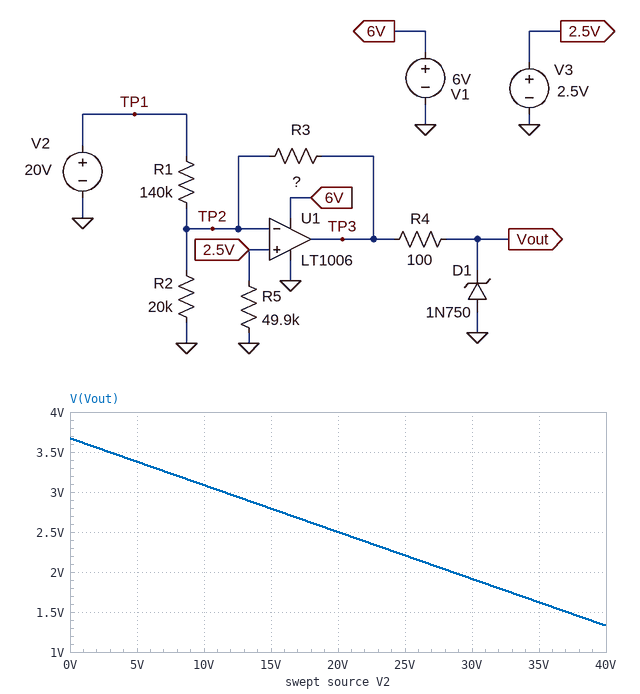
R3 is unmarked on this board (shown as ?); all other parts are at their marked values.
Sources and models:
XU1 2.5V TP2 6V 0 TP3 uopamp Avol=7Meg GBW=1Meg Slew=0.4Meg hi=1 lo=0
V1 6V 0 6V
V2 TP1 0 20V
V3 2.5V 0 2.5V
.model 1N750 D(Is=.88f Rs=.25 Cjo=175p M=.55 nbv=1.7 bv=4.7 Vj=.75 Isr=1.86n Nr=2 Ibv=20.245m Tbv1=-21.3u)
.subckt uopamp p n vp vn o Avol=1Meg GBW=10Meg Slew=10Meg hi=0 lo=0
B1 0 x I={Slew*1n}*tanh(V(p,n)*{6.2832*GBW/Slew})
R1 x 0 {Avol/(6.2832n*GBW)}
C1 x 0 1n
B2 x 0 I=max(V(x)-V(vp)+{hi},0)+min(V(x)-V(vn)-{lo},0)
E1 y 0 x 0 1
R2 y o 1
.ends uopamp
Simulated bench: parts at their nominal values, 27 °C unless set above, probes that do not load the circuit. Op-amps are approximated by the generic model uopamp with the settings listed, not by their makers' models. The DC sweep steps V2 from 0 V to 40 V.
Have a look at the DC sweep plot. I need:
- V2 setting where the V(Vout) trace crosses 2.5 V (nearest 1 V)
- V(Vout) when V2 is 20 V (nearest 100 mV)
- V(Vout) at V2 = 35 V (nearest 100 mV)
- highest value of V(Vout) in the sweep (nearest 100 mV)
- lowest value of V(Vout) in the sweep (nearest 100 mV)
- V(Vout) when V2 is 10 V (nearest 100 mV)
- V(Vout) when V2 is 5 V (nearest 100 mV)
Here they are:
20 V
2.5 V
1.6 V
3.7 V
1.3 V
3.1 V
3.4 V
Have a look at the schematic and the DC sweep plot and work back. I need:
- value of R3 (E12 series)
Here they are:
8.2 kΩ
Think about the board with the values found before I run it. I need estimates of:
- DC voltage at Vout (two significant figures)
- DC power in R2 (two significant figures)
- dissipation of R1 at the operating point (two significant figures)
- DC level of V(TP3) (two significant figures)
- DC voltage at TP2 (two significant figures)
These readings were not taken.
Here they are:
2.5 V
310 µW
2.2 mW
2.5 V
2.5 V
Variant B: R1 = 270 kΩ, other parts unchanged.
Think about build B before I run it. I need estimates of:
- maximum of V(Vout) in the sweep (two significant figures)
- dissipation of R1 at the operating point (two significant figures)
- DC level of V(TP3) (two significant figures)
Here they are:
3.6 V
1.1 mW
3.0 V
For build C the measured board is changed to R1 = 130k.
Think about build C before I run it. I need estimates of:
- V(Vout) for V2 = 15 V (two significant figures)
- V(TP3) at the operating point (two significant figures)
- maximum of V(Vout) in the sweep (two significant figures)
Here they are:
2.7 V
2.4 V
3.7 V
